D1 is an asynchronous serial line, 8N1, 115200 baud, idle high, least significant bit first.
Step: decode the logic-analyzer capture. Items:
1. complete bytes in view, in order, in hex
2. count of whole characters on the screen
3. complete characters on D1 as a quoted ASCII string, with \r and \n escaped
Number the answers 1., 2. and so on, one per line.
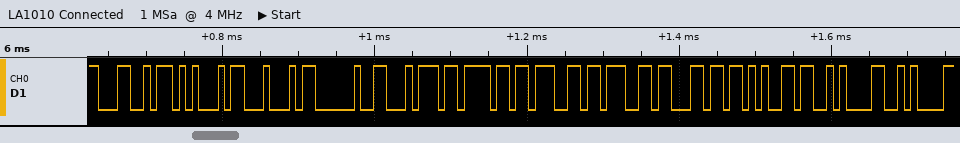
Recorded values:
1. 0x4C 0x45 0x44 0x20 0x74 0x6F 0x67 0x67 0x6C 0x65 0x0A 0x0A
2. 12
3. "LED toggle\n\n"
